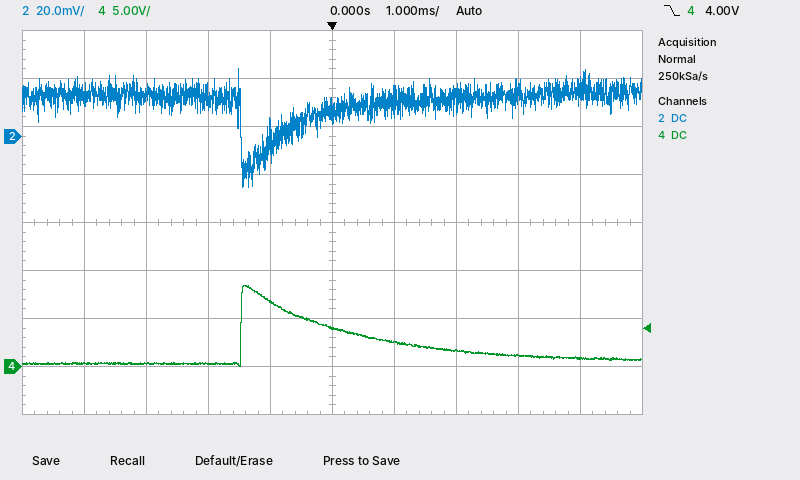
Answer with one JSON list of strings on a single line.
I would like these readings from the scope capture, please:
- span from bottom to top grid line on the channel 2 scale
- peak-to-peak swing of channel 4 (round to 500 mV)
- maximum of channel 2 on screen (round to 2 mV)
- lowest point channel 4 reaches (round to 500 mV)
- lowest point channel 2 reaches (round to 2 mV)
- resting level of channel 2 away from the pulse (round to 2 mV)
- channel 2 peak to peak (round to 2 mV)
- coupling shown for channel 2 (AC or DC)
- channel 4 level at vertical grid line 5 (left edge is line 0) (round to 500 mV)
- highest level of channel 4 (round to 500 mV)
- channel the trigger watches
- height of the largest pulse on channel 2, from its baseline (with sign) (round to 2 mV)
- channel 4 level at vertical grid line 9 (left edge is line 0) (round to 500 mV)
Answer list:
["160 mV", "8.5 V", "28 mV", "0.0 V", "-22 mV", "16 mV", "50 mV", "DC", "4.0 V", "8.5 V", "channel 4", "-38 mV", "1.0 V"]
